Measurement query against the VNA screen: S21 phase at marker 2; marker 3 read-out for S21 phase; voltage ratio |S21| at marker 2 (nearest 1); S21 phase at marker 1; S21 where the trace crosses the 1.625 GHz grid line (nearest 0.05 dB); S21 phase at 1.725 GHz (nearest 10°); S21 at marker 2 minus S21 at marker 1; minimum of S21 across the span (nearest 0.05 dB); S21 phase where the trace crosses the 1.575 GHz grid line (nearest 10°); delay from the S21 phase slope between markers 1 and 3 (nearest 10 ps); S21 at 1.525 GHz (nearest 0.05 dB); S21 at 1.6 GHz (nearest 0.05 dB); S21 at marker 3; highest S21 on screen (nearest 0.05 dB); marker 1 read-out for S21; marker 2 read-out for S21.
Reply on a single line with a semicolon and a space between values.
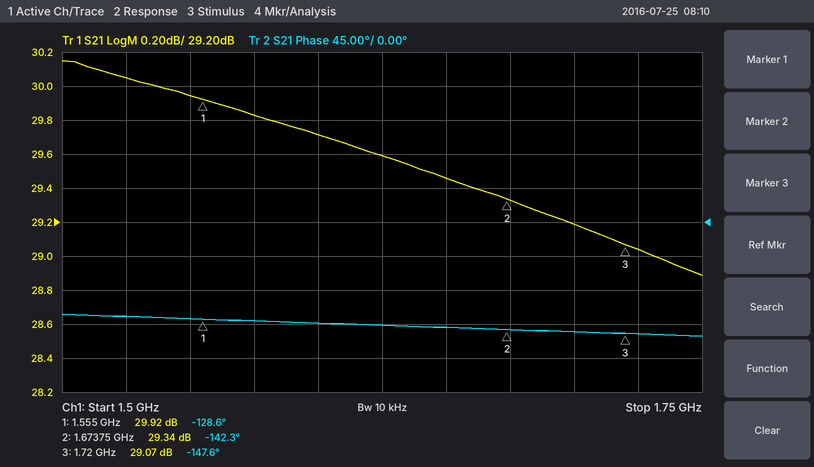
-142.3°; -147.6°; 29; -128.6°; 29.60 dB; -150°; -0.58 dB; 28.90 dB; -130°; 320 ps; 30.05 dB; 29.70 dB; 29.07 dB; 30.15 dB; 29.92 dB; 29.34 dB
